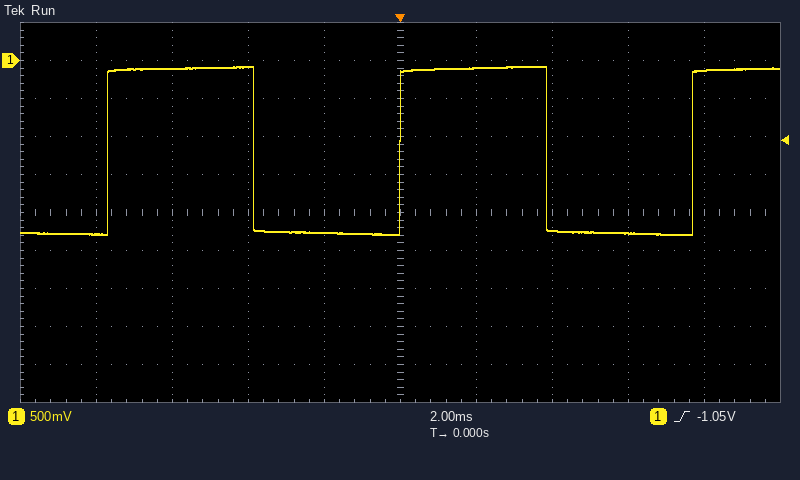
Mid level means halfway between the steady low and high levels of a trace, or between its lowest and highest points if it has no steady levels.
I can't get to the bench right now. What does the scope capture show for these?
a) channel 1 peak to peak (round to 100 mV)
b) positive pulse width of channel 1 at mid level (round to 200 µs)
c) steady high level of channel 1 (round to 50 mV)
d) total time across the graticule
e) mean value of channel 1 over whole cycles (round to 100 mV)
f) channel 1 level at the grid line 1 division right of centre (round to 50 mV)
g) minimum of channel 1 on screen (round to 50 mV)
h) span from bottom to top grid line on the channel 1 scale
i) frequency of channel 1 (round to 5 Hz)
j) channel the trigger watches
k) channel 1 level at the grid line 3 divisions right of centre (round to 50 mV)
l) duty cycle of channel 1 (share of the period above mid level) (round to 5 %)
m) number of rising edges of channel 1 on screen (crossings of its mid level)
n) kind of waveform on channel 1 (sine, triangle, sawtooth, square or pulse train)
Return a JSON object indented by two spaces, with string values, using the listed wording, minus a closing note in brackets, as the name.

{
  "channel 1 peak to peak": "2.20 V",
  "positive pulse width of channel 1 at mid level": "3.8 ms",
  "steady high level of channel 1": "-100 mV",
  "total time across the graticule": "20 ms",
  "mean value of channel 1 over whole cycles": "-1.2 V",
  "channel 1 level at the grid line 1 division right of centre": "-100 mV",
  "minimum of channel 1 on screen": "-2.30 V",
  "span from bottom to top grid line on the channel 1 scale": "5 V",
  "frequency of channel 1": "130 Hz",
  "channel the trigger watches": "channel 1",
  "channel 1 level at the grid line 3 divisions right of centre": "-2.25 V",
  "duty cycle of channel 1 (share of the period above mid level)": "50 %",
  "number of rising edges of channel 1 on screen": "3",
  "kind of waveform on channel 1": "square"
}
